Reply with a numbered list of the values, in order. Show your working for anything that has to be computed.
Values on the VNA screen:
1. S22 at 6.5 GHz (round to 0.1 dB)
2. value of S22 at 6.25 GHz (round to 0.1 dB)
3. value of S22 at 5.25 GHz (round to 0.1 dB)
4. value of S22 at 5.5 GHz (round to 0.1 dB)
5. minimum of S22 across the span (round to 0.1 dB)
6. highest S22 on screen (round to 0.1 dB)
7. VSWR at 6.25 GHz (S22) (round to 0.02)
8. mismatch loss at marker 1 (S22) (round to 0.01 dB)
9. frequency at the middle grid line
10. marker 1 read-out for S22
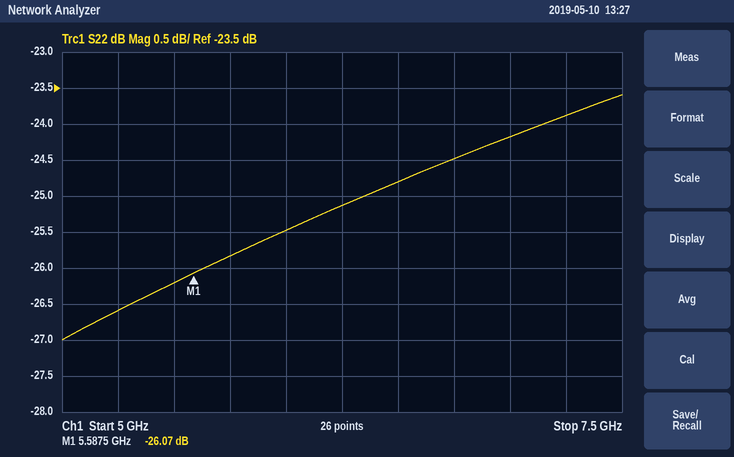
1. -24.8 dB
2. -25.1 dB
3. -26.6 dB
4. -26.2 dB
5. -27.0 dB
6. -23.6 dB
7. |Γ| = 10^(-25.1/20) = 0.0556; VSWR = (1 + 0.0556)/(1 − 0.0556) ≈ 1.12
8. −10 log10(1 − 10^(-26.07/10)) ≈ 0.01 dB
9. 6.25 GHz
10. -26.07 dB
